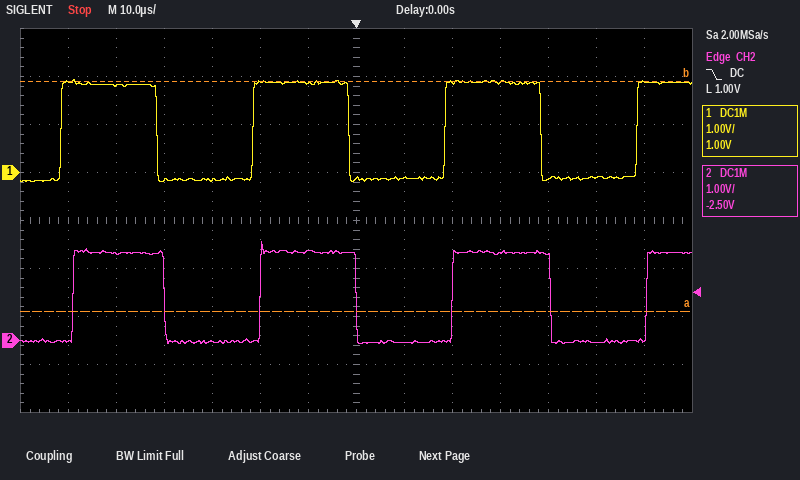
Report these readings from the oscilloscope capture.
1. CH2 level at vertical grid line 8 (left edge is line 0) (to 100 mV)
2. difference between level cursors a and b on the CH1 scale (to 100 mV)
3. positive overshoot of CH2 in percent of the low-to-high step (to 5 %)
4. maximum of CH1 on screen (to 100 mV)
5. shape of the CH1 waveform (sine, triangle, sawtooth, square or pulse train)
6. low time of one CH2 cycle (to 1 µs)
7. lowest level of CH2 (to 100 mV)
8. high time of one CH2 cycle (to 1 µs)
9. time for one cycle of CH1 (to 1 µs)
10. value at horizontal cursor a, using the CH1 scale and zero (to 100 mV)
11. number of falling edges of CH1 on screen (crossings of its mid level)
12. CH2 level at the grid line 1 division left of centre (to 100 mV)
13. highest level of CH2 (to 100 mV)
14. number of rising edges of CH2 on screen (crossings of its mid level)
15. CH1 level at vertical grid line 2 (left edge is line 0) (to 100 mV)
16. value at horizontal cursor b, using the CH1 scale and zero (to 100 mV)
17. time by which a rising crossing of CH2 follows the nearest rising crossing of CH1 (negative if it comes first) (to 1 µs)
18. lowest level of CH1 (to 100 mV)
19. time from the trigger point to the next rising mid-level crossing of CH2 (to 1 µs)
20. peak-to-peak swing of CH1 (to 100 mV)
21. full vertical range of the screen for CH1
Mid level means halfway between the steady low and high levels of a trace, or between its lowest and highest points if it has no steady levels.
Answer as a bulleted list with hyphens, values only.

- 0.0 V
- 4.8 V
- 10 %
- 1.9 V
- square
- 20 µs
- -100 mV
- 20 µs
- 40 µs
- -2.9 V
- 3
- 1.9 V
- 2.1 V
- 4
- 1.8 V
- 1.9 V
- +2 µs
- -200 mV
- 20 µs
- 2.1 V
- 8 V
